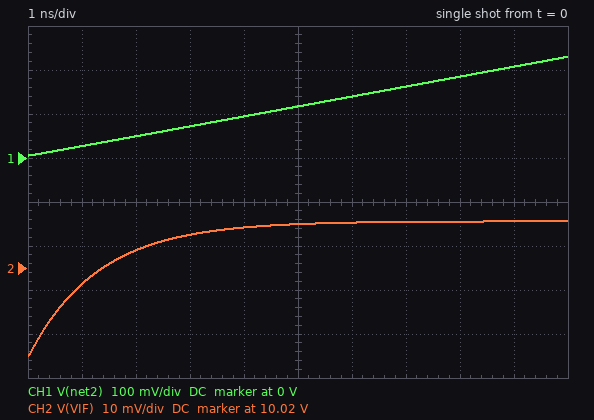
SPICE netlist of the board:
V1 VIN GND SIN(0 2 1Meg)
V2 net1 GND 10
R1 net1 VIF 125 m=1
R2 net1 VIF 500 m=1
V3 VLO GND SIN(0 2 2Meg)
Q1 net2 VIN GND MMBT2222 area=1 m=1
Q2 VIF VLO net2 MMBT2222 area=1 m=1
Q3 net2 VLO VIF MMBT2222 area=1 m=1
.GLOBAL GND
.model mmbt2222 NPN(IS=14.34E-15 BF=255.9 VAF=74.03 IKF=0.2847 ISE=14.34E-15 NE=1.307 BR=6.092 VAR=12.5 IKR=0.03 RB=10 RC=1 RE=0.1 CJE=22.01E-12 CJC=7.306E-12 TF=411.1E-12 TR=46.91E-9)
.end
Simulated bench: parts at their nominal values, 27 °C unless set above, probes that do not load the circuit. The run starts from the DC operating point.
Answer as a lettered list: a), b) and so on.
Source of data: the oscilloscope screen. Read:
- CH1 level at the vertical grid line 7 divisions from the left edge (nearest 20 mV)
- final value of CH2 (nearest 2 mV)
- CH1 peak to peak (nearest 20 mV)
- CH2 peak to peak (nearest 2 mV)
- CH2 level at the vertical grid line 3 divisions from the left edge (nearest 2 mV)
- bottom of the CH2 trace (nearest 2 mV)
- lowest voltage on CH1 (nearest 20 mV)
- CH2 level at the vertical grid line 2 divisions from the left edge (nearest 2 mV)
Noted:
a) 160 mV
b) 10.030 V
c) 220 mV
d) 30 mV
e) 10.028 V
f) 10.000 V
g) 0 V
h) 10.024 V
